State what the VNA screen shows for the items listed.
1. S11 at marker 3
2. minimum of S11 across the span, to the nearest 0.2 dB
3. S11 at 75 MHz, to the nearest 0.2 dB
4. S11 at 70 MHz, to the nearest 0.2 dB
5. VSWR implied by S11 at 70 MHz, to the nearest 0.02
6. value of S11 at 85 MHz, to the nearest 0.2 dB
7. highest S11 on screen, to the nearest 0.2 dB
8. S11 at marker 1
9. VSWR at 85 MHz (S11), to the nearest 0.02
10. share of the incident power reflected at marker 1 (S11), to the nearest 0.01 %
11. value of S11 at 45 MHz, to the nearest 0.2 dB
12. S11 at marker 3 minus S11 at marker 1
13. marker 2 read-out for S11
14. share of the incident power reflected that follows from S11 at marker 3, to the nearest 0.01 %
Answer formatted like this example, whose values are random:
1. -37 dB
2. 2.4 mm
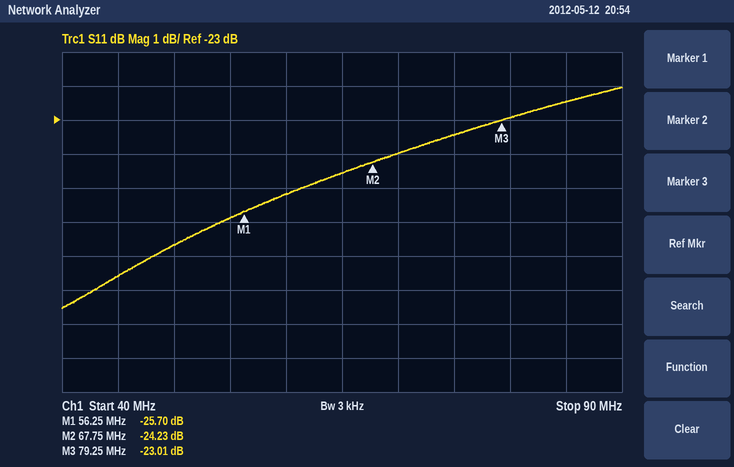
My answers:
1. -23.01 dB
2. -28.6 dB
3. -23.4 dB
4. -24.0 dB
5. 1.14
6. -22.4 dB
7. -22.0 dB
8. -25.70 dB
9. 1.16
10. 0.27 %
11. -27.6 dB
12. 2.69 dB
13. -24.23 dB
14. 0.50 %
